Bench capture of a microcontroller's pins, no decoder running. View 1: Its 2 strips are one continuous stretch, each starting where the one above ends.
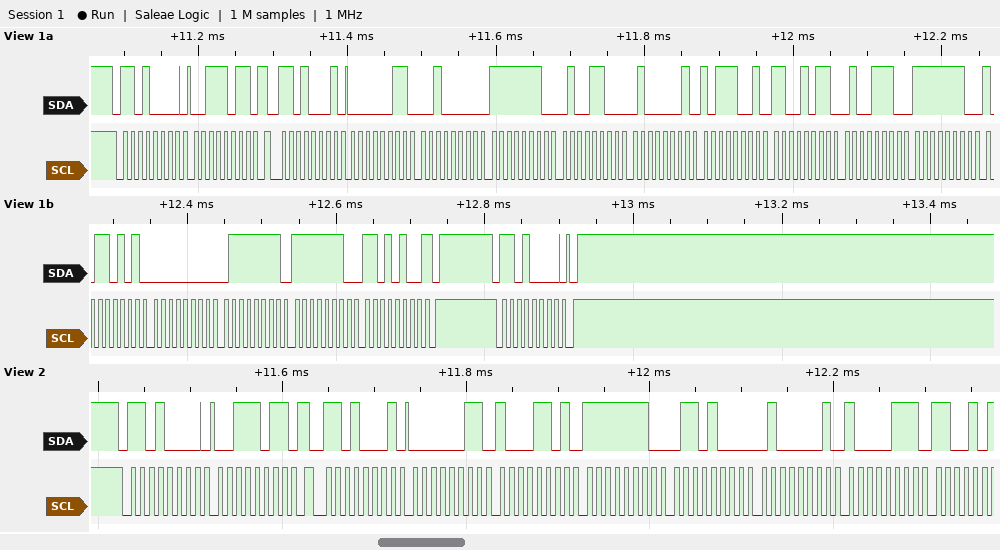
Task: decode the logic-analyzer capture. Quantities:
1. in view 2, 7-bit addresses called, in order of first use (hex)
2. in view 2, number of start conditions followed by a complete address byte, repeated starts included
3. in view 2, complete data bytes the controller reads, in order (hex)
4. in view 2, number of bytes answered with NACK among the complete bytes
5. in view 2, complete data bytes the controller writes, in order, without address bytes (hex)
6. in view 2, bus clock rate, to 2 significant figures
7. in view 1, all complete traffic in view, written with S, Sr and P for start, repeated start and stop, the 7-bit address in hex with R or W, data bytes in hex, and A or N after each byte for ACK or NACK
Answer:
0x68
2
03 8D FE 68 41 87
0
3B
100 kHz
S 68W A 3B A Sr 68R A 03 A 20 A FE A 4C A 41 A B9 A CB A 4E A FE A B5 A 00 A 7F A FE A D4 N P S 68W A P
